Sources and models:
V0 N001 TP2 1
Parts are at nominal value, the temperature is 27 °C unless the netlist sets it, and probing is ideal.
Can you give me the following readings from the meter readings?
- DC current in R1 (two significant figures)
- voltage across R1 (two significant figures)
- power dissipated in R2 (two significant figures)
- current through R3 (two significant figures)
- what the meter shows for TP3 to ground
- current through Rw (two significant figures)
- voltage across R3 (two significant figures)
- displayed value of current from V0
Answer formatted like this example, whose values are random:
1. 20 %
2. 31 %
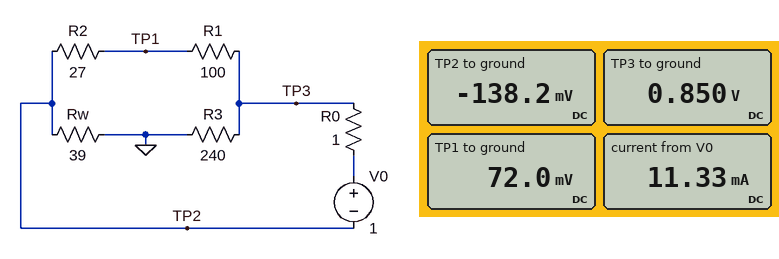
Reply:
1. 7.8 mA
2. 780 mV
3. 1.6 mW
4. 3.5 mA
5. 0.850 V
6. 3.5 mA
7. 850 mV
8. 11.33 mA
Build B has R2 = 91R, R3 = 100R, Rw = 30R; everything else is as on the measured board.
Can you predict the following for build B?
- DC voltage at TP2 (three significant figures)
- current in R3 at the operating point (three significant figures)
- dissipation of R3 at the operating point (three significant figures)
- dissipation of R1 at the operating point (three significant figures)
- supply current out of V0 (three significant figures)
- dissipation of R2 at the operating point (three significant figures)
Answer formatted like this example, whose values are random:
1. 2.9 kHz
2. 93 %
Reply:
1. -228 mV
2. 7.59 mA
3. 5.77 mW
4. 2.67 mW
5. 12.8 mA
6. 2.43 mW
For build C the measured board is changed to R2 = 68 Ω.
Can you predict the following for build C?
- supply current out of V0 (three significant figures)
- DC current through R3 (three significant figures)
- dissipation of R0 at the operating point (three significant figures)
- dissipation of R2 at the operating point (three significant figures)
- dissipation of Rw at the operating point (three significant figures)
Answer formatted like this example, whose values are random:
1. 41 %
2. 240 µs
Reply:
1. 9.45 mA
2. 3.55 mA
3. 89.2 µW
4. 2.36 mW
5. 492 µW
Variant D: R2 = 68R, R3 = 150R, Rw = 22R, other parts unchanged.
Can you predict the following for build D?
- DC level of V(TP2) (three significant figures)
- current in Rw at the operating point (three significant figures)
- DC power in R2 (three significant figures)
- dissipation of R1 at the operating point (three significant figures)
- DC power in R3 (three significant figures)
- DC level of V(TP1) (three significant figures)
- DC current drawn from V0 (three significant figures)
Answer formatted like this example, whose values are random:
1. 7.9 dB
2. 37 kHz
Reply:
1. -126 mV
2. 5.75 mA
3. 2.35 mW
4. 3.46 mW
5. 4.95 mW
6. 274 mV
7. 11.6 mA
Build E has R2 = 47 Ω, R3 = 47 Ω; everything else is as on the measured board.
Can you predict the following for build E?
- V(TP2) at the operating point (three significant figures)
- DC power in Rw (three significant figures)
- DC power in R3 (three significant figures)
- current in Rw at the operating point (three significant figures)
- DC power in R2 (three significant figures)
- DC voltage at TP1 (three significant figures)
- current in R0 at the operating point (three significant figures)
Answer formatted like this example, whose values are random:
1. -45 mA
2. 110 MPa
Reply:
1. -445 mV
2. 5.08 mW
3. 6.13 mW
4. 11.4 mA
5. 2.10 mW
6. -131 mV
7. 18.1 mA
